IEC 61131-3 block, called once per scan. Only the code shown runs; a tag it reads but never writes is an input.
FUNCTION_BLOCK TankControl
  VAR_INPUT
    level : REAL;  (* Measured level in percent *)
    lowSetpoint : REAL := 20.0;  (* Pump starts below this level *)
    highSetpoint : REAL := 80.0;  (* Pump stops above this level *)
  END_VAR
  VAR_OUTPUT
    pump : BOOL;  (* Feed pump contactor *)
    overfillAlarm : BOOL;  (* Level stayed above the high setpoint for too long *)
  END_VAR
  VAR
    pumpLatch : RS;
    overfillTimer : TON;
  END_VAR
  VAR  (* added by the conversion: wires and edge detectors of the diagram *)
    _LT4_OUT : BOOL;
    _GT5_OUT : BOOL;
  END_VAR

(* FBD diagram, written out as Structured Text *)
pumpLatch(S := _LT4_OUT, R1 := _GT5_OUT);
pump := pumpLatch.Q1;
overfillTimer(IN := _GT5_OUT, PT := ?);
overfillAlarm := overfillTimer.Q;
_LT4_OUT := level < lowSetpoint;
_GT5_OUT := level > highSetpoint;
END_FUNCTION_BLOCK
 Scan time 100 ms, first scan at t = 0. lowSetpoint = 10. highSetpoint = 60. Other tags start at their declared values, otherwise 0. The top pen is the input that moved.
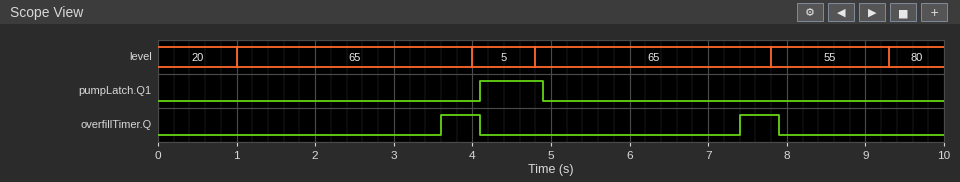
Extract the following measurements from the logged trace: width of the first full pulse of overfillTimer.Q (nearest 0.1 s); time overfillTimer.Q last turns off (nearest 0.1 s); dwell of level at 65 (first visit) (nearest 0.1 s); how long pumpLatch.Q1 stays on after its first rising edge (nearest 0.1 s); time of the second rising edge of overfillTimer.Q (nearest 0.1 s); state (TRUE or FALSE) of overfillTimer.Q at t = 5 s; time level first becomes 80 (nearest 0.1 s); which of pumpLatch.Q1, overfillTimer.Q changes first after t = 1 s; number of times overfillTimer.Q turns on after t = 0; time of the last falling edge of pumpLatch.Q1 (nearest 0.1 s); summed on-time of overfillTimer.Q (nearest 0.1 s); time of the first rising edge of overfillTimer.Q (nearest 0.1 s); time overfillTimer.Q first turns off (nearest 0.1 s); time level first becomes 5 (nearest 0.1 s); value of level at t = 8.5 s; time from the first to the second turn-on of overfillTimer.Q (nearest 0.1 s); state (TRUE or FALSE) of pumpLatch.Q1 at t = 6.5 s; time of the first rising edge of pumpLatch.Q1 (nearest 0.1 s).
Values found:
0.5 s
7.9 s
3.0 s
0.8 s
7.4 s
FALSE
9.3 s
overfillTimer.Q
2
4.9 s
1.0 s
3.6 s
4.1 s
4.0 s
55
3.8 s
FALSE
4.1 s
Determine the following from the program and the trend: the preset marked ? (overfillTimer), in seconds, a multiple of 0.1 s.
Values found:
2.5 s
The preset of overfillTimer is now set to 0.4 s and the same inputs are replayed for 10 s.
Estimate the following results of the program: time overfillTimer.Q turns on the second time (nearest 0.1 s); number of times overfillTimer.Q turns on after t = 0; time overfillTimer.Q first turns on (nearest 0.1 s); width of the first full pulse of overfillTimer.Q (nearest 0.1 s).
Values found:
5.3 s
3
1.5 s
2.6 s
